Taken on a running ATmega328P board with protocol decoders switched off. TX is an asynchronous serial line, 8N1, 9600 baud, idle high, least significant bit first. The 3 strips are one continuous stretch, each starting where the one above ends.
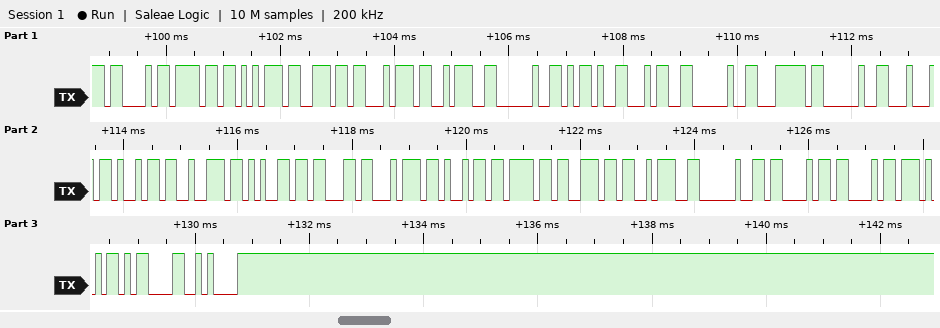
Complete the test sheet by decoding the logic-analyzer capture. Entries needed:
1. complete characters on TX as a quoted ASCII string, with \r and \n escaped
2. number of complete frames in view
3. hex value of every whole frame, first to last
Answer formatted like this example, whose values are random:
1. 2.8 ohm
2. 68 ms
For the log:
1. "Count: -4 | Direction: CCW\r\n"
2. 28
3. 43 6F 75 6E 74 3A 20 2D 34 20 7C 20 44 69 72 65 63 74 69 6F 6E 3A 20 43 43 57 0D 0A
